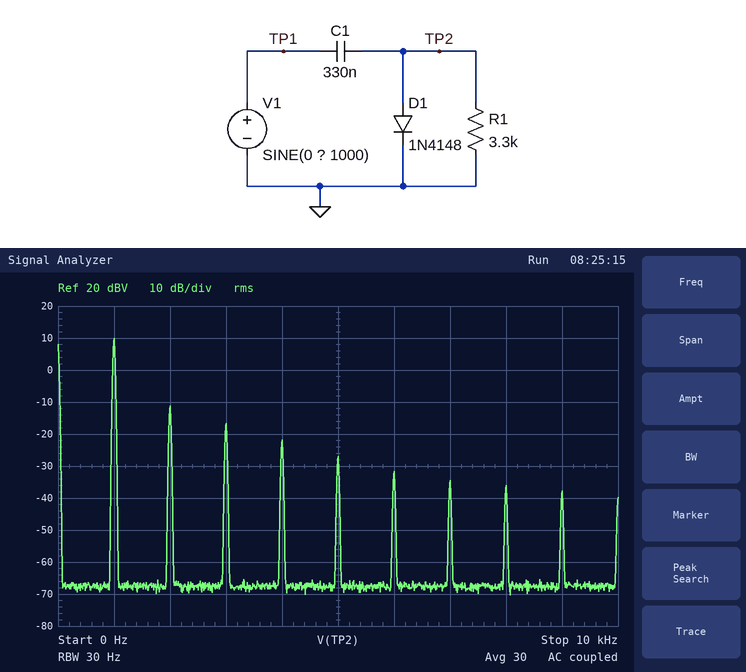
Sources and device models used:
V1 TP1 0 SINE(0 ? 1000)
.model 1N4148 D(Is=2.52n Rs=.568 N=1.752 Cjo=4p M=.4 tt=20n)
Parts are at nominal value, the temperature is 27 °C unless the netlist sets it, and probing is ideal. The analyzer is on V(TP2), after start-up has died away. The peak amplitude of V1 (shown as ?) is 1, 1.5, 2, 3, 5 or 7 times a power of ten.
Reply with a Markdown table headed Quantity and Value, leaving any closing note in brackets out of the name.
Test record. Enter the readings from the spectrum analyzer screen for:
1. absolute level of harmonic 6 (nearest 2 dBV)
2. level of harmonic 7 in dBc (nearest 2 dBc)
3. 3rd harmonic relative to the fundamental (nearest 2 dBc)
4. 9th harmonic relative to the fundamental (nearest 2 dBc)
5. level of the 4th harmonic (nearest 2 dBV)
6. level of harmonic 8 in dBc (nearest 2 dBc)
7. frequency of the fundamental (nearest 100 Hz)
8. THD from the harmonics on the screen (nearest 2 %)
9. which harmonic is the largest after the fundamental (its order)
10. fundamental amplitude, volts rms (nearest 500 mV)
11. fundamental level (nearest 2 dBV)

| Quantity | Value |
|---|---|
| absolute level of harmonic 6 | -32 dBV |
| level of harmonic 7 in dBc | -44 dBc |
| 3rd harmonic relative to the fundamental | -26 dBc |
| 9th harmonic relative to the fundamental | -48 dBc |
| level of the 4th harmonic | -22 dBV |
| level of harmonic 8 in dBc | -46 dBc |
| frequency of the fundamental | 1.0 kHz |
| THD from the harmonics on the screen | 10 % |
| which harmonic is the largest after the fundamental | 2 |
| fundamental amplitude, volts rms | 3.0 V |
| fundamental level | 10 dBV |
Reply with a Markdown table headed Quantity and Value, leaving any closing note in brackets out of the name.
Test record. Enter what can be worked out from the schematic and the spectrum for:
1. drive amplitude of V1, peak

| Quantity | Value |
|---|---|
| drive amplitude of V1, peak | 5 V |
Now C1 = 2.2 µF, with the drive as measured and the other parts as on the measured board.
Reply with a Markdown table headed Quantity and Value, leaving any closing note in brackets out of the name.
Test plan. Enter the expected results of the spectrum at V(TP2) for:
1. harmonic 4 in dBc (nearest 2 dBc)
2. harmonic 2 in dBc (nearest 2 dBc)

| Quantity | Value |
|---|---|
| harmonic 4 in dBc | -42 dBc |
| harmonic 2 in dBc | -36 dBc |
